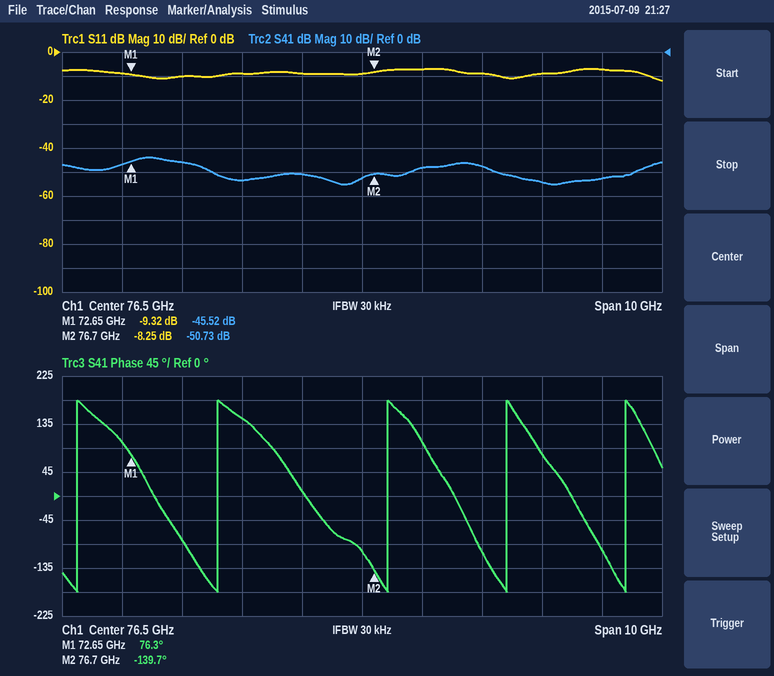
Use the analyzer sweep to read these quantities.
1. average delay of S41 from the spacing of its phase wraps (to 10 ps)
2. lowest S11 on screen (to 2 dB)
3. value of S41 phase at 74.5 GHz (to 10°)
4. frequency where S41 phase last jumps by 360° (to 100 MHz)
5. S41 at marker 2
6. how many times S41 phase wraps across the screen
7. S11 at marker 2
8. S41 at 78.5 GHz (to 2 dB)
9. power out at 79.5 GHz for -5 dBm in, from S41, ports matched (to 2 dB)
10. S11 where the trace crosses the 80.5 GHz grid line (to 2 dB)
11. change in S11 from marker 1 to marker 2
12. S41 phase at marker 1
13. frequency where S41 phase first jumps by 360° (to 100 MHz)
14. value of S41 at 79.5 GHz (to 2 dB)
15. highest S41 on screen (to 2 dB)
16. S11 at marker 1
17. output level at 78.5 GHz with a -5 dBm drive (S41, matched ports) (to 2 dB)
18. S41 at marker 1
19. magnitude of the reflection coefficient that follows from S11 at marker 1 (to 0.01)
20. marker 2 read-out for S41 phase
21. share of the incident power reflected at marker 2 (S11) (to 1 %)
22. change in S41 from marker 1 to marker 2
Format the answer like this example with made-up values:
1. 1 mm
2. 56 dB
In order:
1. 440 ps
2. -12 dB
3. 150°
4. 80.9 GHz
5. -50.73 dB
6. 5
7. -8.25 dB
8. -48 dB
9. -60 dBm
10. -8 dB
11. 1.07 dB
12. 76.3°
13. 71.8 GHz
14. -54 dB
15. -44 dB
16. -9.32 dB
17. -52 dBm
18. -45.52 dB
19. 0.34
20. -139.7°
21. 15 %
22. -5.21 dB
